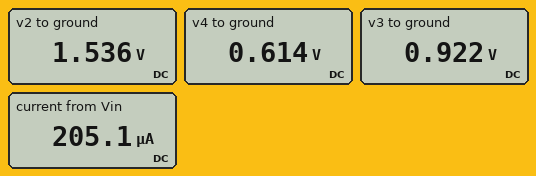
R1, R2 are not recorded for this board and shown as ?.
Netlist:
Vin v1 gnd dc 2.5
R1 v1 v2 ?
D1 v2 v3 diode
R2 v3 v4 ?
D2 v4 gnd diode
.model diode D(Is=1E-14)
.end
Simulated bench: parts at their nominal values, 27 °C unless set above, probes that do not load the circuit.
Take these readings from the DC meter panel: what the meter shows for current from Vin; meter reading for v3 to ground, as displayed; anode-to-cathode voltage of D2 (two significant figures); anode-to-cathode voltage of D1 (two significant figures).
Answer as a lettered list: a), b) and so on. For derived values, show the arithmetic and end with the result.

a) 205.1 µA
b) 0.922 V
c) 614 mV = 610 mV
d) 1.536 V - 922 mV = 610 mV
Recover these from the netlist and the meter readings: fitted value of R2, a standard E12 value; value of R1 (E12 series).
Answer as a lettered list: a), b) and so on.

a) 1.5 kΩ
b) 4.7 kΩ
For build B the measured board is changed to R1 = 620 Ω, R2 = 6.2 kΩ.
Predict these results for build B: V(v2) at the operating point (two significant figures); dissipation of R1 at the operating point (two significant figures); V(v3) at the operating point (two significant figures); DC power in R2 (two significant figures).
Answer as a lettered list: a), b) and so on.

a) 2.4 V
b) 22 µW
c) 1.8 V
d) 220 µW
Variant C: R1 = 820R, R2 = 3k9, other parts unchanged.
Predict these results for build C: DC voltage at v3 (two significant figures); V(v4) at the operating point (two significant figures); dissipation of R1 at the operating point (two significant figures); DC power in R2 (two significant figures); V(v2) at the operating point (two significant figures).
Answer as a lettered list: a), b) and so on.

a) 1.7 V
b) 620 mV
c) 58 µW
d) 280 µW
e) 2.3 V
